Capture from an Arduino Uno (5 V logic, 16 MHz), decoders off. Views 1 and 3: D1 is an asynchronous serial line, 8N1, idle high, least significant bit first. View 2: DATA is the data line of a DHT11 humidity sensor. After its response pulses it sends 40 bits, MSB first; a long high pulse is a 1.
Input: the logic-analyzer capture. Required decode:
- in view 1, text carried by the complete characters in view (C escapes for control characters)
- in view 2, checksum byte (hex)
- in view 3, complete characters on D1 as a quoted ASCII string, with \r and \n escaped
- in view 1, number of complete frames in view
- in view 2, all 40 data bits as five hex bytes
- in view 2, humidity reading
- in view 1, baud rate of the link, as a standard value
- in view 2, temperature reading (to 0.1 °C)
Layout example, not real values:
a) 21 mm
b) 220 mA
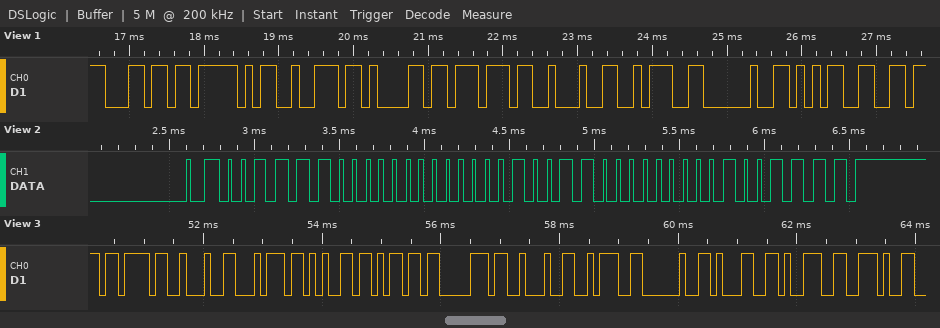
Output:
a) "l_raw\": 5"
b) 0x4F
c) "{\"temp\": 19."
d) 9
e) 3C 00 13 00 4F
f) 60 %
g) 9600 baud
h) 19.0 °C
